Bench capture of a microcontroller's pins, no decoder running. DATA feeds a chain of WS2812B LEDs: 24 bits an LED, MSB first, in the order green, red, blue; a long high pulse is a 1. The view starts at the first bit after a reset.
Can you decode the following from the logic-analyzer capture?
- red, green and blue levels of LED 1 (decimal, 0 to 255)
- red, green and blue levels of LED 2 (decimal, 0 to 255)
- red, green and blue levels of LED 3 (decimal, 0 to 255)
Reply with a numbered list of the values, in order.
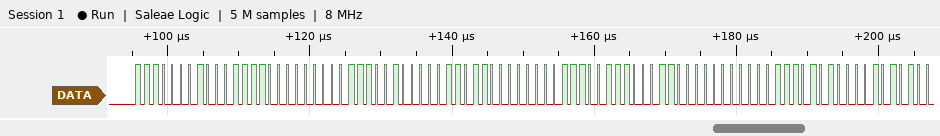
1. 30, 225, 0
2. 27, 228, 0
3. 24, 231, 0
